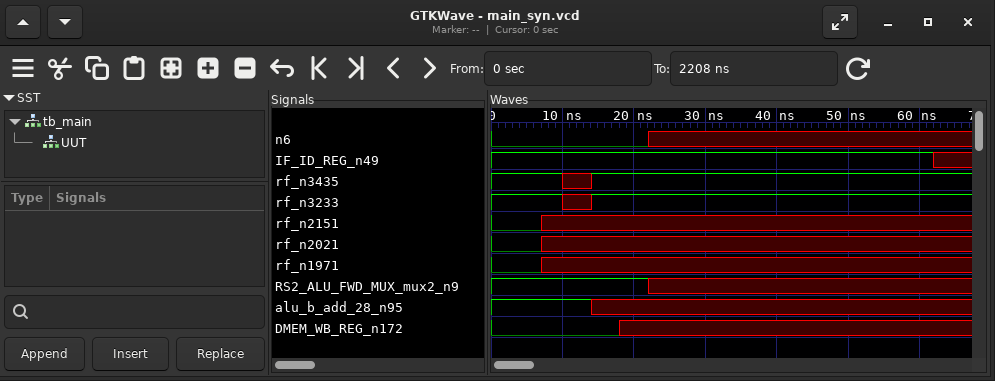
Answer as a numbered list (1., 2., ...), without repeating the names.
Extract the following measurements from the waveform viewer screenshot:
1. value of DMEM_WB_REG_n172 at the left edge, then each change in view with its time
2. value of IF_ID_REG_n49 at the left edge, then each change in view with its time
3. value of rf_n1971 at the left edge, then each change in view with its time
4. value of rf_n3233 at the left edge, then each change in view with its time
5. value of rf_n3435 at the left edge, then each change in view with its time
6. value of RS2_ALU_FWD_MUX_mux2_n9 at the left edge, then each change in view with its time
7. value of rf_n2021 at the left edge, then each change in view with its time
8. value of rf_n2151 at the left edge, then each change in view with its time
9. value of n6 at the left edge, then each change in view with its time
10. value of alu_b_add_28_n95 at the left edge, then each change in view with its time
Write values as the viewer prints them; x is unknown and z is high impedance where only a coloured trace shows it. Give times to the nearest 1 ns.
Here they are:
1. 0, x at 18 ns
2. 1, x at 62 ns
3. 0, x at 7 ns
4. 1, x at 10 ns, 1 at 14 ns
5. 1, x at 10 ns, 1 at 14 ns
6. 1, x at 22 ns
7. 0, x at 7 ns
8. 0, x at 7 ns
9. 0, x at 22 ns
10. 1, x at 14 ns
